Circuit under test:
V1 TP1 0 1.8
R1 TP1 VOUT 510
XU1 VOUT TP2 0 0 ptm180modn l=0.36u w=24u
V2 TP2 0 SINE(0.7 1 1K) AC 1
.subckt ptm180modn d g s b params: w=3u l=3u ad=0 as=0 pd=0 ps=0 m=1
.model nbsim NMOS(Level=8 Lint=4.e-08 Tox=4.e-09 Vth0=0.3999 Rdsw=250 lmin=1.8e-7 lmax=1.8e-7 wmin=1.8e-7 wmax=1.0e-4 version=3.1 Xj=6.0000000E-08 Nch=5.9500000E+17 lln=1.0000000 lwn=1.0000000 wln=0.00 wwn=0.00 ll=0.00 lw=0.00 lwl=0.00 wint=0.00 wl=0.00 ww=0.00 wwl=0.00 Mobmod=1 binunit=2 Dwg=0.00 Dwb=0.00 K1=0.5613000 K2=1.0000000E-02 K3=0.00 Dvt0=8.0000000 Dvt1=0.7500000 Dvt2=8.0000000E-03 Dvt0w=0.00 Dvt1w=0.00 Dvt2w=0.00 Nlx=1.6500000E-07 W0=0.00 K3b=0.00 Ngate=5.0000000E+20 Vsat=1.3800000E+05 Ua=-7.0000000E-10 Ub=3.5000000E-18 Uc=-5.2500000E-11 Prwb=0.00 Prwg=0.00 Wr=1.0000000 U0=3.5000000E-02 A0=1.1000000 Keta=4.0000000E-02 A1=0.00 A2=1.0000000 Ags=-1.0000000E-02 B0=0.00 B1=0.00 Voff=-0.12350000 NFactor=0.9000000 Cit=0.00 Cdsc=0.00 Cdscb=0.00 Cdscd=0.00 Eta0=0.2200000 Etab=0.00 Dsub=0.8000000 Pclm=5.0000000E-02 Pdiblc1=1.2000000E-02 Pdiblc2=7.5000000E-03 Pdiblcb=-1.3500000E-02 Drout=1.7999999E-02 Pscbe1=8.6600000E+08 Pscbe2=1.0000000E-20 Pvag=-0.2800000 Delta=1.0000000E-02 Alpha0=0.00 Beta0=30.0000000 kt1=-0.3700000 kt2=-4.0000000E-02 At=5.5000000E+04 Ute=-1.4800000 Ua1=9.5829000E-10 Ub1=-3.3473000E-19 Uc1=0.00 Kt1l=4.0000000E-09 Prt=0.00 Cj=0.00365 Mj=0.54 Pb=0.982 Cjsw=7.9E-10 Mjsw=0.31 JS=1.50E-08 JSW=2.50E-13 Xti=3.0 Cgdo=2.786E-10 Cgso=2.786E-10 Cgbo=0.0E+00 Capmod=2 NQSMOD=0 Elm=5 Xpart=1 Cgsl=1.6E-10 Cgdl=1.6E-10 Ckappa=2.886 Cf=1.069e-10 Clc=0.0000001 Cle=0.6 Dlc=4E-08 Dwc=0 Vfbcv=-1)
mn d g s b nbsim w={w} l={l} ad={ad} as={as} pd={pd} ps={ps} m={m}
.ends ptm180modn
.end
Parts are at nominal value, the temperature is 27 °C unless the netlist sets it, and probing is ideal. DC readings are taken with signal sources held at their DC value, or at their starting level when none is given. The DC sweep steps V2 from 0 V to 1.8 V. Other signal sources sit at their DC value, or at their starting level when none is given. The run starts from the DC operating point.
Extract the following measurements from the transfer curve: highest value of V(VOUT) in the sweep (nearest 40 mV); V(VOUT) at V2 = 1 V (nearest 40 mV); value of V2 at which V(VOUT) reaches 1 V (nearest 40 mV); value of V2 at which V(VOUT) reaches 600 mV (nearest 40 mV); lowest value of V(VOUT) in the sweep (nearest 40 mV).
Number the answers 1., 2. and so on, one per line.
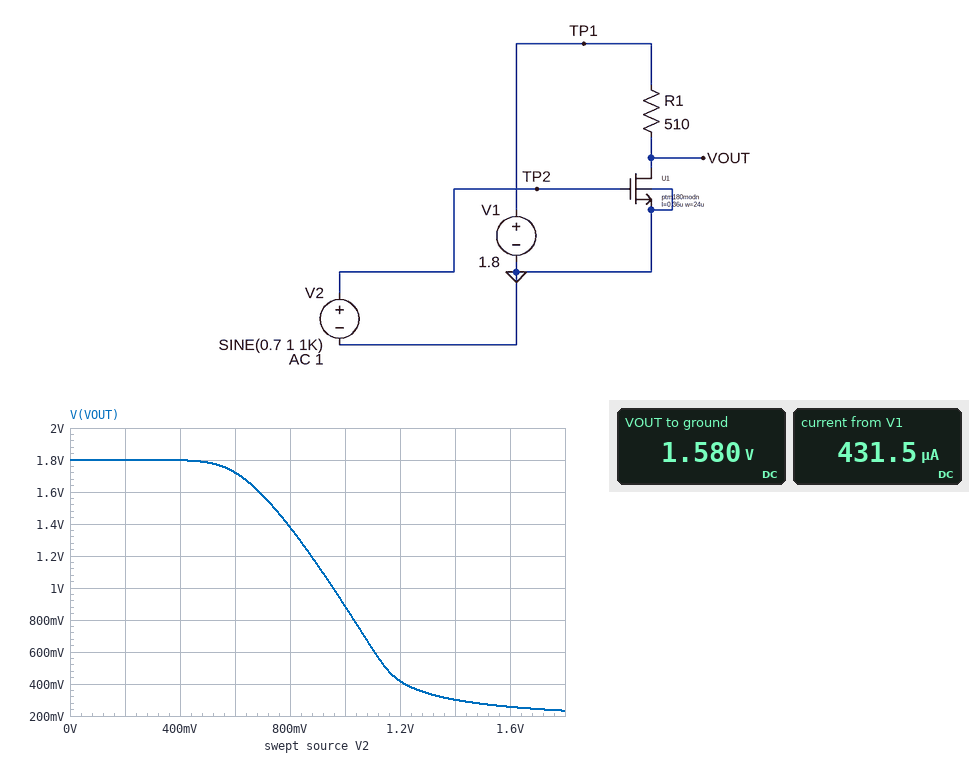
1. 1.80 V
2. 880 mV
3. 960 mV
4. 1.12 V
5. 240 mV
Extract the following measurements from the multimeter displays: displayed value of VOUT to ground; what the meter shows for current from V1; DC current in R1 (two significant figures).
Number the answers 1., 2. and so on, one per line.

1. 1.580 V
2. 431.5 µA
3. 430 µA
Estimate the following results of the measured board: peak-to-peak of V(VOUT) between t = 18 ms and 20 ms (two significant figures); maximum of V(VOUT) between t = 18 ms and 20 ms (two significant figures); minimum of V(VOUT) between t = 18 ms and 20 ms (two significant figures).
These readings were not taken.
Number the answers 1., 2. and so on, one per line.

1. 1.6 V
2. 1.8 V
3. 240 mV
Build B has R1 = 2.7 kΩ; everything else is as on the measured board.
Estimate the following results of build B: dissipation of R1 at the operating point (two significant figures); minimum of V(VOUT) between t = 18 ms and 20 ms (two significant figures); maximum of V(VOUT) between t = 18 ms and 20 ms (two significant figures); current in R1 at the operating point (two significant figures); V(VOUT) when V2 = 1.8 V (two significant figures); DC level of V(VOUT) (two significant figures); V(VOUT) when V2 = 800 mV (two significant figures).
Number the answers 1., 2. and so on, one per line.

1. 380 µW
2. 45 mV
3. 1.8 V
4. 370 µA
5. 44 mV
6. 790 mV
7. 180 mV
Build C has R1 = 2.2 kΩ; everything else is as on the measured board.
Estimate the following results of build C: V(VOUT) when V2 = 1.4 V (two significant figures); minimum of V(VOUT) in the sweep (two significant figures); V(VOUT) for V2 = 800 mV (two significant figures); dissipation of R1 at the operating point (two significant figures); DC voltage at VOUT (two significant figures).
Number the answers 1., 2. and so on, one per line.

1. 65 mV
2. 54 mV
3. 290 mV
4. 330 µW
5. 950 mV
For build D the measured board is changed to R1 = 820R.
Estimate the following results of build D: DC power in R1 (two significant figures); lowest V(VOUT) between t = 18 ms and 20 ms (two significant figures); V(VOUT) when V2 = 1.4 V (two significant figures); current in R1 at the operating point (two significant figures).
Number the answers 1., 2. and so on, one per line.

1. 150 µW
2. 150 mV
3. 180 mV
4. 420 µA
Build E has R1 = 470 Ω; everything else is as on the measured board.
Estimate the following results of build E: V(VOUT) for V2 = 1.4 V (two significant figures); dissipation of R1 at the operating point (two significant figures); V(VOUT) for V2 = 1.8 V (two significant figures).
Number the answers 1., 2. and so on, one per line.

1. 330 mV
2. 88 µW
3. 250 mV
